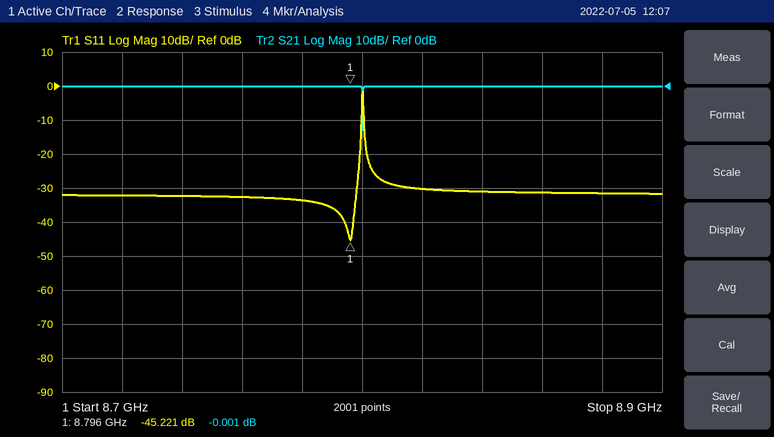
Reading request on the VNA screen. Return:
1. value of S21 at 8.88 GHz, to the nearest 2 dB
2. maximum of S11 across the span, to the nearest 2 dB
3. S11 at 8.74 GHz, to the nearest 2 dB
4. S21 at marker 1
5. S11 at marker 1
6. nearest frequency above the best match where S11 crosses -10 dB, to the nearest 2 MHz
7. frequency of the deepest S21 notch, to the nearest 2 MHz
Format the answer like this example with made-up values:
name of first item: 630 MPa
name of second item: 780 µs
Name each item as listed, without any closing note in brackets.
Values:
value of S21 at 8.88 GHz, to the nearest 2 dB: 0 dB
maximum of S11 across the span, to the nearest 2 dB: -2 dB
S11 at 8.74 GHz, to the nearest 2 dB: -32 dB
S21 at marker 1: -0.001 dB
S11 at marker 1: -45.221 dB
nearest frequency above the best match where S11 crosses -10 dB, to the nearest 2 MHz: 8.800 GHz
frequency of the deepest S21 notch, to the nearest 2 MHz: 8.800 GHz
